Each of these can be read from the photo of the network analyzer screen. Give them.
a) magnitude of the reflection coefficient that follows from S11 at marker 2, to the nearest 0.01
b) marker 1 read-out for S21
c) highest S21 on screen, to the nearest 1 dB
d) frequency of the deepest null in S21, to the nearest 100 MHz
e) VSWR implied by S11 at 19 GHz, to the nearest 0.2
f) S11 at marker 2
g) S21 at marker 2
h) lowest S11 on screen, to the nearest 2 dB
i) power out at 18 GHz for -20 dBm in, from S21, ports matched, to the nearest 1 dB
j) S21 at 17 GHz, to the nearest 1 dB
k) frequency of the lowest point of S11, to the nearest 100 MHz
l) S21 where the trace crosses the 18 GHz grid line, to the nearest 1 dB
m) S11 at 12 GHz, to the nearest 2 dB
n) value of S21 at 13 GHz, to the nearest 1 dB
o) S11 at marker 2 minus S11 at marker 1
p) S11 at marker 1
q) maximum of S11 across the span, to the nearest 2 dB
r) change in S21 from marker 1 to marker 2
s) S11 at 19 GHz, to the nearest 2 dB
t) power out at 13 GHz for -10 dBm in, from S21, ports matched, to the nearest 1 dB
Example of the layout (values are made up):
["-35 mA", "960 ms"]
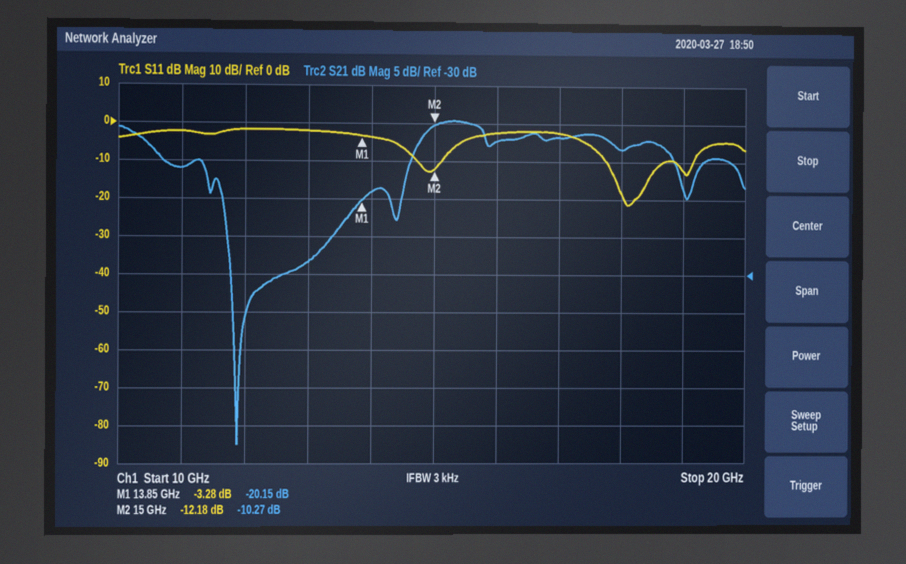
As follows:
["0.25", "-20.15 dB", "-10 dB", "11.9 GHz", "1.6", "-12.18 dB", "-10.27 dB", "-22 dB", "-33 dBm", "-12 dB", "18.1 GHz", "-13 dB", "-2 dB", "-28 dB", "-8.90 dB", "-3.28 dB", "-2 dB", "9.88 dB", "-12 dB", "-38 dBm"]
